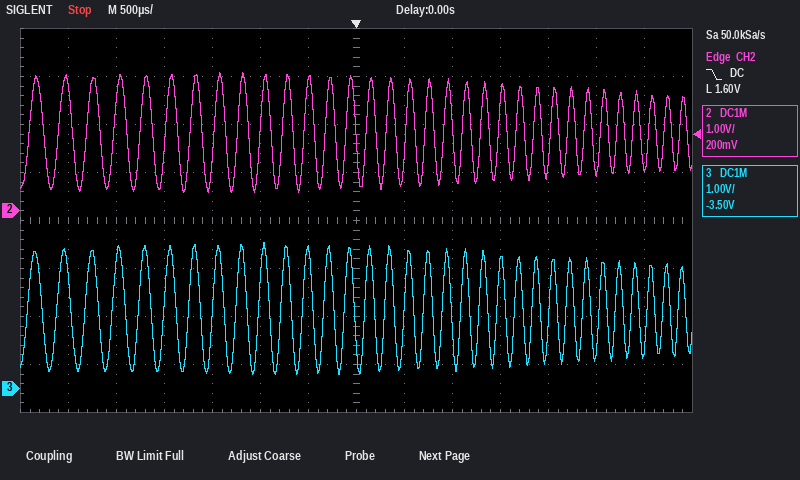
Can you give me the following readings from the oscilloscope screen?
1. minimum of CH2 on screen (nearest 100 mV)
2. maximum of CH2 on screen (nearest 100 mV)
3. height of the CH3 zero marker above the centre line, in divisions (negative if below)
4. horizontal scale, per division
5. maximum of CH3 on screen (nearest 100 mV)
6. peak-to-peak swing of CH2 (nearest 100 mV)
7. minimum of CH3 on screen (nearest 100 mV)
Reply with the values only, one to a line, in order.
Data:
400 mV
2.9 V
-3.5 div
500 µs
3.0 V
2.5 V
300 mV
